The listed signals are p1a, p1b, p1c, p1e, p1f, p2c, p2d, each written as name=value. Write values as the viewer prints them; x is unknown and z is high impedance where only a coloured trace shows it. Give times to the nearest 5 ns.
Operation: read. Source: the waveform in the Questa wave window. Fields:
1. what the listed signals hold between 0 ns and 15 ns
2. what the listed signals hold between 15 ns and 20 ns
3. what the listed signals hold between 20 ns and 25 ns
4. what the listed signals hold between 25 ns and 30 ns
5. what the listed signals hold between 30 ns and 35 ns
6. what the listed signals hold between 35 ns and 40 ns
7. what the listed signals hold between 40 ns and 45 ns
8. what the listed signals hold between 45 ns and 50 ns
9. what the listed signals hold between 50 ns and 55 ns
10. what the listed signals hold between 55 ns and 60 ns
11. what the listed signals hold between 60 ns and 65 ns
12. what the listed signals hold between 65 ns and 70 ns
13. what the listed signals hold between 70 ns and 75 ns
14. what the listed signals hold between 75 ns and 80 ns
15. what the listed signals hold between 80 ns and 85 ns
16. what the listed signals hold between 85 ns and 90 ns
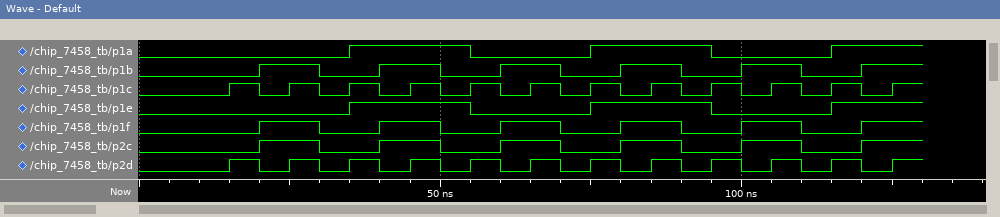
p1a=0, p1b=0, p1c=0, p1e=0, p1f=0, p2c=0, p2d=0
p1a=0, p1b=0, p1c=1, p1e=0, p1f=0, p2c=0, p2d=1
p1a=0, p1b=1, p1c=0, p1e=0, p1f=1, p2c=1, p2d=0
p1a=0, p1b=1, p1c=1, p1e=0, p1f=1, p2c=1, p2d=1
p1a=0, p1b=0, p1c=0, p1e=0, p1f=0, p2c=0, p2d=0
p1a=1, p1b=0, p1c=1, p1e=1, p1f=0, p2c=0, p2d=1
p1a=1, p1b=1, p1c=0, p1e=1, p1f=1, p2c=1, p2d=0
p1a=1, p1b=1, p1c=1, p1e=1, p1f=1, p2c=1, p2d=1
p1a=1, p1b=0, p1c=0, p1e=1, p1f=0, p2c=0, p2d=0
p1a=0, p1b=0, p1c=1, p1e=0, p1f=0, p2c=0, p2d=1
p1a=0, p1b=1, p1c=0, p1e=0, p1f=1, p2c=1, p2d=0
p1a=0, p1b=1, p1c=1, p1e=0, p1f=1, p2c=1, p2d=1
p1a=0, p1b=0, p1c=0, p1e=0, p1f=0, p2c=0, p2d=0
p1a=1, p1b=0, p1c=1, p1e=1, p1f=0, p2c=0, p2d=1
p1a=1, p1b=1, p1c=0, p1e=1, p1f=1, p2c=1, p2d=0
p1a=1, p1b=1, p1c=1, p1e=1, p1f=1, p2c=1, p2d=1
